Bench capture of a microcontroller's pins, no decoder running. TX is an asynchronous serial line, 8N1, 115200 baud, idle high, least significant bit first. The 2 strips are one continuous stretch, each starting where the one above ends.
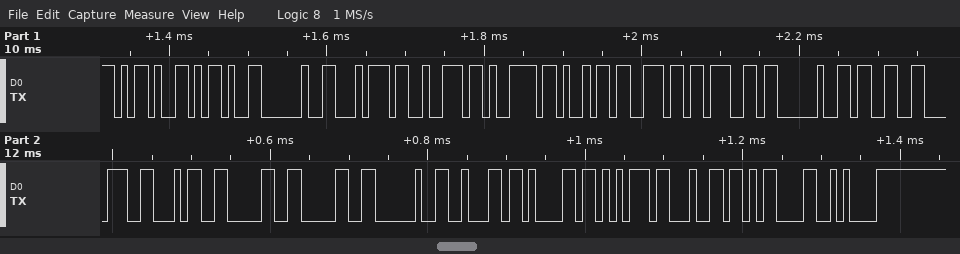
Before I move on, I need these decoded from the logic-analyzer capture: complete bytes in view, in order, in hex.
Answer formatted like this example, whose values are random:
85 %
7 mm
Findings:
0x2D 0x2D 0x20 0x74 0x72 0x79 0x69 0x6E 0x67 0x20 0x33 0x38 0x34 0x30 0x30 0x20 0x62 0x61 0x75 0x64 0x0D 0x0A
